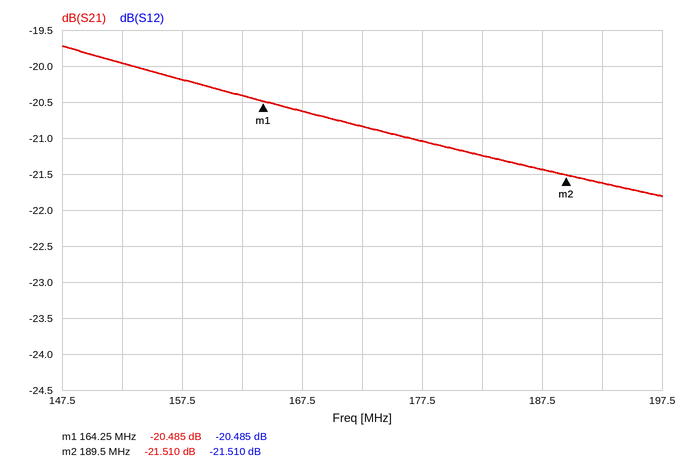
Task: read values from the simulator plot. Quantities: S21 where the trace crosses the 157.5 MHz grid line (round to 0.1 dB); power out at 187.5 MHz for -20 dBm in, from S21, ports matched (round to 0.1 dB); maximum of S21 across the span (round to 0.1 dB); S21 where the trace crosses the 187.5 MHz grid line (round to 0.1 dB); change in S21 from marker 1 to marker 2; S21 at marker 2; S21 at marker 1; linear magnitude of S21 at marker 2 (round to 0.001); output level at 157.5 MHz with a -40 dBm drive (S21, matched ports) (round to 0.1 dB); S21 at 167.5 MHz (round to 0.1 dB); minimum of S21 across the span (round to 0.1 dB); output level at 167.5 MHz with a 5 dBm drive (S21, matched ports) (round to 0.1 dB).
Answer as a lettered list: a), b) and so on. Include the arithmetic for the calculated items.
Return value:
a) -20.2 dB
b) -20 dBm + (-21.4 dB) = -41.4 dBm
c) -19.7 dB
d) -21.4 dB
e) -21.51 − (-20.485) = -1.025 dB
f) -21.510 dB
g) -20.485 dB
h) 10^(-21.51/20) ≈ 0.084
i) -40 dBm + (-20.2 dB) = -60.2 dBm
j) -20.6 dB
k) -21.8 dB
l) 5 dBm + (-20.6 dB) = -15.6 dBm
